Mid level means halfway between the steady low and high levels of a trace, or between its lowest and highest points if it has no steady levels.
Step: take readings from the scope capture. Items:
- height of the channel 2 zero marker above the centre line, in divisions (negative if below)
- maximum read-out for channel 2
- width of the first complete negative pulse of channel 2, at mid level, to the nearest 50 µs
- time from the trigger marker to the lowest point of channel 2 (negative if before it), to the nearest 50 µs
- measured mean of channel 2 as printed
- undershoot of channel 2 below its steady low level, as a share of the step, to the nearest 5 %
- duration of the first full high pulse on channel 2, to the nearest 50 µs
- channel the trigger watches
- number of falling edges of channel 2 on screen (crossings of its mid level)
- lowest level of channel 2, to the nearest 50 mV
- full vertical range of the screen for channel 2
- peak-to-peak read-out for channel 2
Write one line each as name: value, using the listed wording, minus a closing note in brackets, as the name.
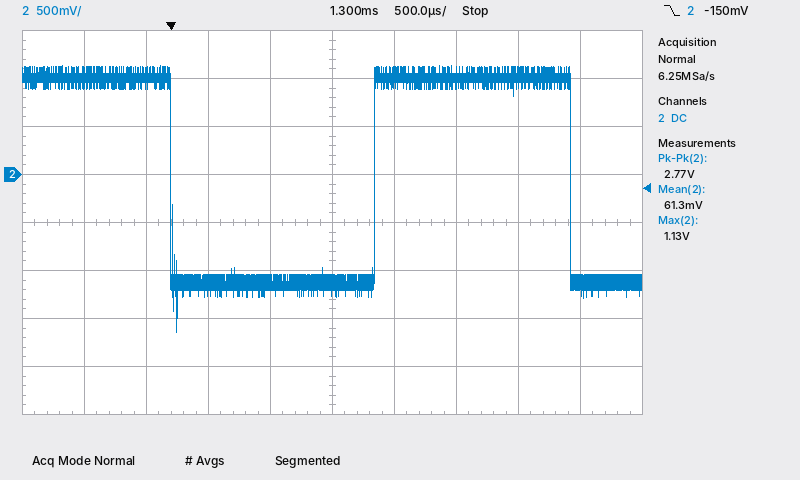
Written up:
height of the channel 2 zero marker above the centre line, in divisions: +1.0 div
maximum read-out for channel 2: 1.13 V
width of the first complete negative pulse of channel 2, at mid level, to the nearest 50 µs: 1.65 ms
time from the trigger marker to the lowest point of channel 2 (negative if before it), to the nearest 50 µs: +50 µs
measured mean of channel 2 as printed: 61.3 mV
undershoot of channel 2 below its steady low level, as a share of the step, to the nearest 5 %: 25 %
duration of the first full high pulse on channel 2, to the nearest 50 µs: 1.60 ms
channel the trigger watches: channel 2
number of falling edges of channel 2 on screen: 2
lowest level of channel 2, to the nearest 50 mV: -1.65 V
full vertical range of the screen for channel 2: 4 V
peak-to-peak read-out for channel 2: 2.77 V
